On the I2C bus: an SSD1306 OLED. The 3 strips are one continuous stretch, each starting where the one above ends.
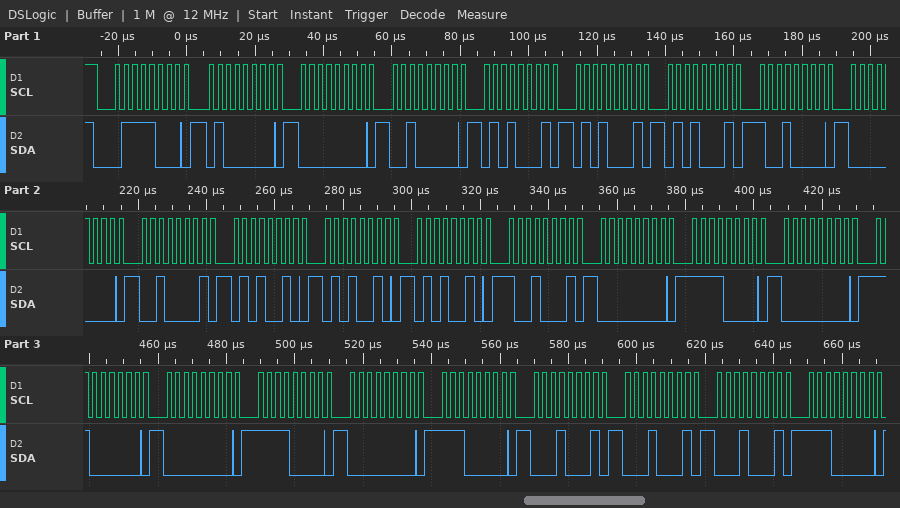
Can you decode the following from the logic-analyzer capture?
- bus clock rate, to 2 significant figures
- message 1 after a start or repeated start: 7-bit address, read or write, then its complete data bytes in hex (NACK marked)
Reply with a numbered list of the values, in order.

1. 400 kHz
2. 0x3C write: 40 00 20 51 51 51 90 00 21 52 52 52 91 00 F0 00 C0 00 F0 00 E0 11 11 11 E0
